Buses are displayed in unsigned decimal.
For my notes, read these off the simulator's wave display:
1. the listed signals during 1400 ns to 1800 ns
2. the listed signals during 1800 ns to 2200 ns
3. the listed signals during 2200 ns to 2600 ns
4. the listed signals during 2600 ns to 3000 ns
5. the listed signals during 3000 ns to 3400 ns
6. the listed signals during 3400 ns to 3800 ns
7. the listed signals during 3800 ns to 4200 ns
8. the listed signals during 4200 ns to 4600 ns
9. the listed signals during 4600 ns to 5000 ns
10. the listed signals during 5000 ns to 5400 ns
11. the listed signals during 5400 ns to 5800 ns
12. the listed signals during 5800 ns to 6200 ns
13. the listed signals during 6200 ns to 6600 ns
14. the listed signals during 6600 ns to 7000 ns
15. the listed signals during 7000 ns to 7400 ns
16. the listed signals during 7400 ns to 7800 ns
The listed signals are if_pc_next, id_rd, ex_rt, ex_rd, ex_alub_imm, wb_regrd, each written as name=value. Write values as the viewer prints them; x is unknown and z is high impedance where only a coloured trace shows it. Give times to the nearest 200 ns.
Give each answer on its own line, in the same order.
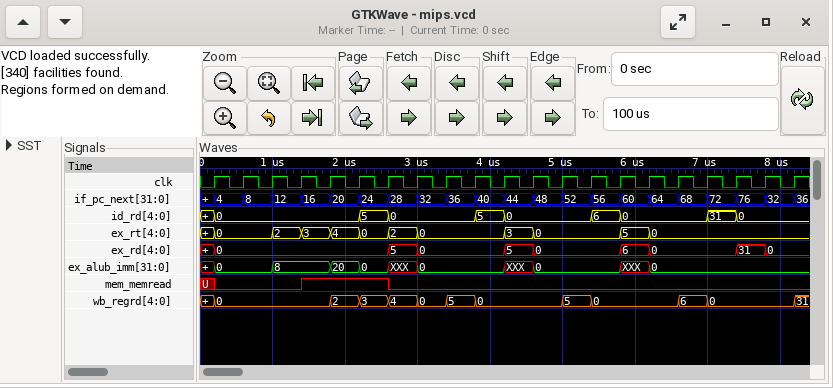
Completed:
if_pc_next=16, id_rd=0, ex_rt=3, ex_rd=0, ex_alub_imm=8, wb_regrd=0
if_pc_next=20, id_rd=0, ex_rt=4, ex_rd=0, ex_alub_imm=20, wb_regrd=2
if_pc_next=24, id_rd=5, ex_rt=0, ex_rd=0, ex_alub_imm=0, wb_regrd=3
if_pc_next=28, id_rd=0, ex_rt=2, ex_rd=5, ex_alub_imm=XXX, wb_regrd=4
if_pc_next=32, id_rd=0, ex_rt=0, ex_rd=0, ex_alub_imm=0, wb_regrd=0
if_pc_next=36, id_rd=0, ex_rt=0, ex_rd=0, ex_alub_imm=0, wb_regrd=5
if_pc_next=40, id_rd=5, ex_rt=0, ex_rd=0, ex_alub_imm=0, wb_regrd=0
if_pc_next=44, id_rd=0, ex_rt=3, ex_rd=5, ex_alub_imm=XXX, wb_regrd=0
if_pc_next=48, id_rd=0, ex_rt=0, ex_rd=0, ex_alub_imm=0, wb_regrd=0
if_pc_next=52, id_rd=0, ex_rt=0, ex_rd=0, ex_alub_imm=0, wb_regrd=5
if_pc_next=56, id_rd=6, ex_rt=0, ex_rd=0, ex_alub_imm=0, wb_regrd=0
if_pc_next=60, id_rd=0, ex_rt=5, ex_rd=6, ex_alub_imm=XXX, wb_regrd=0
if_pc_next=64, id_rd=0, ex_rt=0, ex_rd=0, ex_alub_imm=0, wb_regrd=0
if_pc_next=68, id_rd=0, ex_rt=0, ex_rd=0, ex_alub_imm=0, wb_regrd=6
if_pc_next=72, id_rd=31, ex_rt=0, ex_rd=0, ex_alub_imm=0, wb_regrd=0
if_pc_next=76, id_rd=0, ex_rt=0, ex_rd=31, ex_alub_imm=0, wb_regrd=0
